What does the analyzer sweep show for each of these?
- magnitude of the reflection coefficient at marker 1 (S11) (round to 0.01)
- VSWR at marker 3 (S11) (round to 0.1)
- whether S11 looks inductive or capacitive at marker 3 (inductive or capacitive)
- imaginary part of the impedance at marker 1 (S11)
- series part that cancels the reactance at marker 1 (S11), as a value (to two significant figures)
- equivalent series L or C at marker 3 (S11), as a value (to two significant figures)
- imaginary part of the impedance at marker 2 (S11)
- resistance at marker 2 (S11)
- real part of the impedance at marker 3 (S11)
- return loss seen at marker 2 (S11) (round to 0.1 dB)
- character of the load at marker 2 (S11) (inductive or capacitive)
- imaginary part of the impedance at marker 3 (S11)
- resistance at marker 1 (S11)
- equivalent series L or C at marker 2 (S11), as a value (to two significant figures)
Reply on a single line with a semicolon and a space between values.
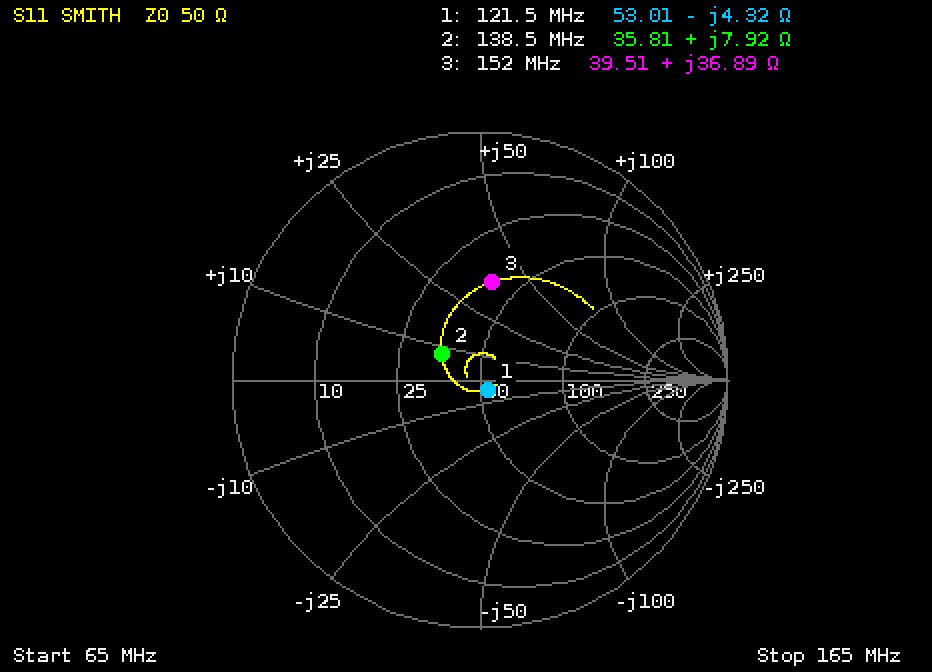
0.05; 2.3; inductive; -4.32 Ω; 5.7 nH; 39 nH; +7.92 Ω; 35.81 Ω; 39.51 Ω; 14.5 dB; inductive; +36.89 Ω; 53.01 Ω; 9.1 nH
